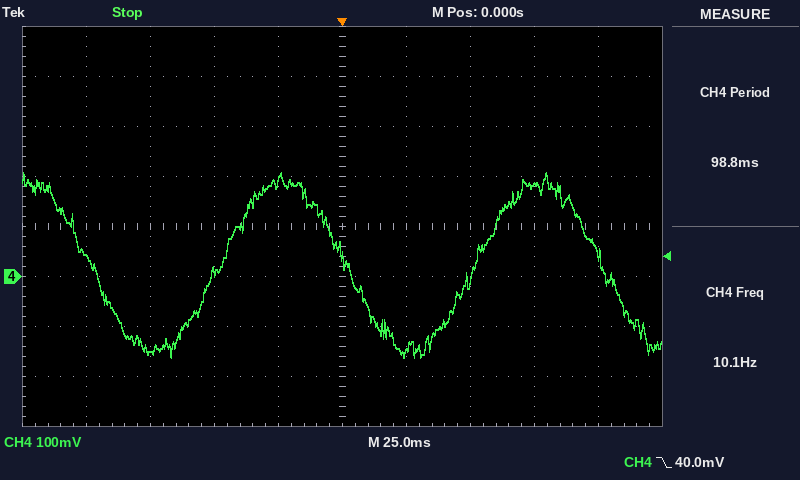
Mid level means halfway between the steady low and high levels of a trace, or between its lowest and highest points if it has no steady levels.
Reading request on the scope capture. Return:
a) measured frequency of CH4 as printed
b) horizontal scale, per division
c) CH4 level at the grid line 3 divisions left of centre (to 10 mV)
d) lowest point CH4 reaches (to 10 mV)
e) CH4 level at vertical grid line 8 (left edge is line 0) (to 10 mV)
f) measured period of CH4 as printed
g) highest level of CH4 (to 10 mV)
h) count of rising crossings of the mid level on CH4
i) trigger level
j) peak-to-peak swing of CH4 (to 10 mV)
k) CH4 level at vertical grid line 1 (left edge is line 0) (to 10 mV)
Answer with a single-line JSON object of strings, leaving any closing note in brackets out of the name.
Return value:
{"measured frequency of CH4 as printed": "10.1 Hz", "horizontal scale, per division": "25 ms", "CH4 level at the grid line 3 divisions left of centre": "-150 mV", "lowest point CH4 reaches": "-160 mV", "CH4 level at vertical grid line 8 (left edge is line 0)": "180 mV", "measured period of CH4 as printed": "98.8 ms", "highest level of CH4": "210 mV", "count of rising crossings of the mid level on CH4": "2", "trigger level": "40.0 mV", "peak-to-peak swing of CH4": "370 mV", "CH4 level at vertical grid line 1 (left edge is line 0)": "40 mV"}
